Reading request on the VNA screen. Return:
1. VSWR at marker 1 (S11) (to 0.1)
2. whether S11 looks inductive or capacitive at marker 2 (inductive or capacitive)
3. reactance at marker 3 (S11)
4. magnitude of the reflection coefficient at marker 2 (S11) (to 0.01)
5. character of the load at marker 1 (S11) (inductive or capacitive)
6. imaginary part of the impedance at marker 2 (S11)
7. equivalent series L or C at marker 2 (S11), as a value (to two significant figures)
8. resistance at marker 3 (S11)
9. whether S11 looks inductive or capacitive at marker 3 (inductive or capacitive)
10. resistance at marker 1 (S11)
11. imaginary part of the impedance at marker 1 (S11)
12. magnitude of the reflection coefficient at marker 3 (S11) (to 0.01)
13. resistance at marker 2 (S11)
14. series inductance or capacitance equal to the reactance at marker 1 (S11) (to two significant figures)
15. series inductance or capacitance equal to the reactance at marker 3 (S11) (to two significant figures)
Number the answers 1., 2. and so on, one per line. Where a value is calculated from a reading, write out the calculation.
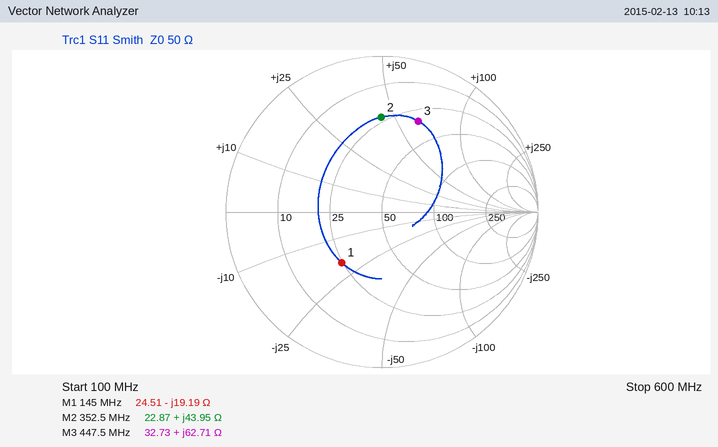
1. 2.4
2. inductive
3. +62.71 Ω
4. 0.61
5. capacitive
6. +43.95 Ω
7. L = 43.95 Ω/(2π × 352.5 MHz) ≈ 20 nH
8. 32.73 Ω
9. inductive
10. 24.51 Ω
11. -19.19 Ω
12. 0.63
13. 22.87 Ω
14. C = 1/(2π × 145 MHz × 19.19 Ω) ≈ 57 pF
15. L = 62.71 Ω/(2π × 447.5 MHz) ≈ 22 nH
